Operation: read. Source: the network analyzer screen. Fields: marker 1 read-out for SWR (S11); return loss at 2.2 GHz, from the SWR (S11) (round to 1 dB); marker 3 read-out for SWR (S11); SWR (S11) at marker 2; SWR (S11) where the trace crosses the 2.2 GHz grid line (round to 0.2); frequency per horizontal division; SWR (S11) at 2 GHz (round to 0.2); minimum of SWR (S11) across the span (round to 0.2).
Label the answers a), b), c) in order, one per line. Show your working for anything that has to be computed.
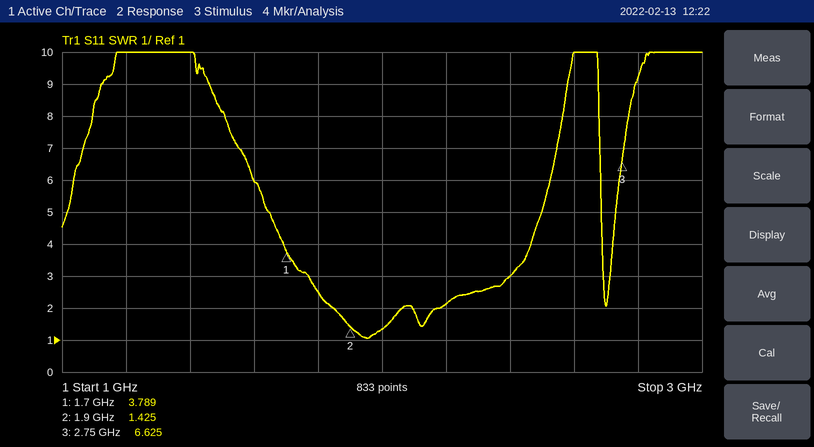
a) 3.789
b) −20 log10((2.2 − 1)/(2.2 + 1)) ≈ 9 dB
c) 6.625
d) 1.425
e) 2.2
f) 200 MHz
g) 1.4
h) 1.0
